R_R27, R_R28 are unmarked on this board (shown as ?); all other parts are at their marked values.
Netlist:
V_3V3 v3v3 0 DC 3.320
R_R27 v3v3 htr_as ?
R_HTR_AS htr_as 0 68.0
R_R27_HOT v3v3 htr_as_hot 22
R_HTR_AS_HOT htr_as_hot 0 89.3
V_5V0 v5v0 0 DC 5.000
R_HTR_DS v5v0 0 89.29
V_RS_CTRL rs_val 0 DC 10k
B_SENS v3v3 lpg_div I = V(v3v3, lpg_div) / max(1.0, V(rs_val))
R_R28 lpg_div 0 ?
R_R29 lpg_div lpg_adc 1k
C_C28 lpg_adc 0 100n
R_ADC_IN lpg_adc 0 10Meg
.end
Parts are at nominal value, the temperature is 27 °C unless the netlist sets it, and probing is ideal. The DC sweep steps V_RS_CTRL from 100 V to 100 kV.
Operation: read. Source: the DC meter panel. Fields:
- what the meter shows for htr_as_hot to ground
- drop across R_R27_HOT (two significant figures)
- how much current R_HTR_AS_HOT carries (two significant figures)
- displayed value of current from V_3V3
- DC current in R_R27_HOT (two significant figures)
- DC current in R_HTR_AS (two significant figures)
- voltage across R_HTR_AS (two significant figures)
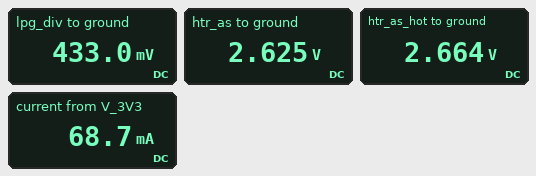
2.664 V
660 mV
30 mA
68.7 mA
30 mA
39 mA
2.6 V
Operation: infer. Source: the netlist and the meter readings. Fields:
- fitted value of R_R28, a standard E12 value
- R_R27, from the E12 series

1.5 kΩ
18 Ω
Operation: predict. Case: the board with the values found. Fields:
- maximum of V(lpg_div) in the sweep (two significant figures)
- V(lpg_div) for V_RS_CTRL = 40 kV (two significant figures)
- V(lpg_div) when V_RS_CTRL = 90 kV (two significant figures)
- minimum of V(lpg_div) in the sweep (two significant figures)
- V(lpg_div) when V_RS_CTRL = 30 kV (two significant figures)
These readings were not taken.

3.1 V
120 mV
54 mV
49 mV
160 mV
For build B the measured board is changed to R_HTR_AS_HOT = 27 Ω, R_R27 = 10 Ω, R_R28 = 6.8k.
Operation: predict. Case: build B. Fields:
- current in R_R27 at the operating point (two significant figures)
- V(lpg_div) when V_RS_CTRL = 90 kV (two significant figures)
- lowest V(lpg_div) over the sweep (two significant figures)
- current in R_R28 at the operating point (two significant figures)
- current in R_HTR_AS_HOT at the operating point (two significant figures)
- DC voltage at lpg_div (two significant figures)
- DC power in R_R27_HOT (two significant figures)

43 mA
230 mV
210 mV
200 µA
68 mA
1.3 V
100 mW
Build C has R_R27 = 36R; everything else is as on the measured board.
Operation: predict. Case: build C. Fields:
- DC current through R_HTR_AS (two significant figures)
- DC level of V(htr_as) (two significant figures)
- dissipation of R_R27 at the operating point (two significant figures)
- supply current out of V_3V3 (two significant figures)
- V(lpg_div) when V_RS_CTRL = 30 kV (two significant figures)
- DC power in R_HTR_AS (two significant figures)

32 mA
2.2 V
37 mW
62 mA
160 mV
69 mW
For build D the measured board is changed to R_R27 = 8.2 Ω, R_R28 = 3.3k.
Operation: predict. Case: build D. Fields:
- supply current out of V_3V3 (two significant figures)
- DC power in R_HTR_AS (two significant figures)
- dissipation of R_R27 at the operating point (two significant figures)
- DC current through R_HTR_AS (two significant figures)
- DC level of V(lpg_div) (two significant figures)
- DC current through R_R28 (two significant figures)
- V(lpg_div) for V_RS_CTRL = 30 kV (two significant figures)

74 mA
130 mW
16 mW
44 mA
820 mV
250 µA
330 mV
